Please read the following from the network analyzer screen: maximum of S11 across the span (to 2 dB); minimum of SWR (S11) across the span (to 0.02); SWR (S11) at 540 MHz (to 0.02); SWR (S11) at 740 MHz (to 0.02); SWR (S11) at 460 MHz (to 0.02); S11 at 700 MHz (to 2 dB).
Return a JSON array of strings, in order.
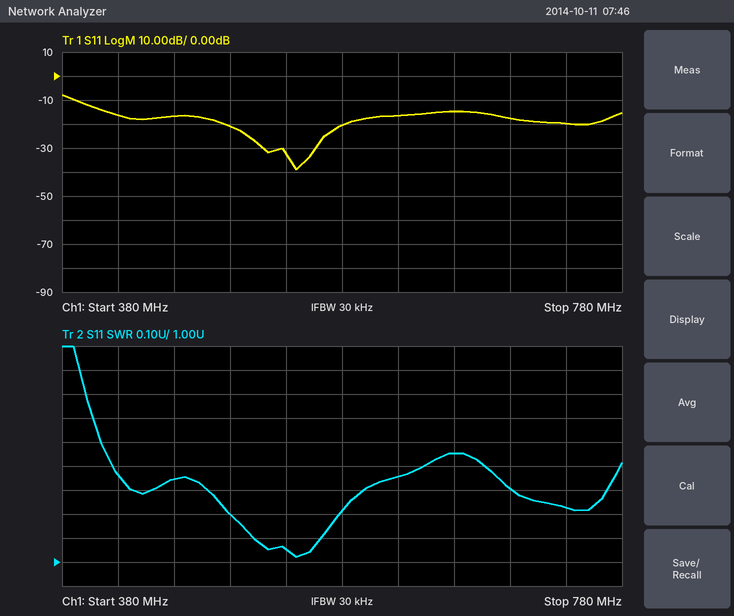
["-8 dB", "1.02", "1.06", "1.22", "1.34", "-18 dB"]
